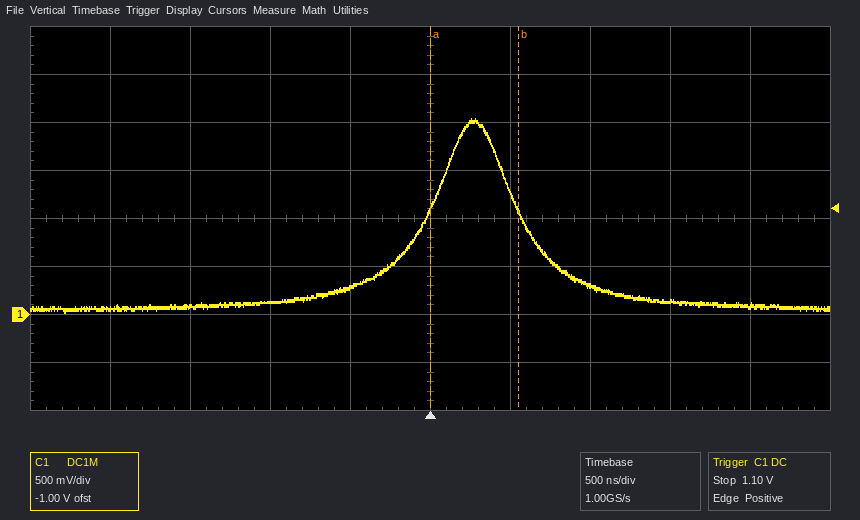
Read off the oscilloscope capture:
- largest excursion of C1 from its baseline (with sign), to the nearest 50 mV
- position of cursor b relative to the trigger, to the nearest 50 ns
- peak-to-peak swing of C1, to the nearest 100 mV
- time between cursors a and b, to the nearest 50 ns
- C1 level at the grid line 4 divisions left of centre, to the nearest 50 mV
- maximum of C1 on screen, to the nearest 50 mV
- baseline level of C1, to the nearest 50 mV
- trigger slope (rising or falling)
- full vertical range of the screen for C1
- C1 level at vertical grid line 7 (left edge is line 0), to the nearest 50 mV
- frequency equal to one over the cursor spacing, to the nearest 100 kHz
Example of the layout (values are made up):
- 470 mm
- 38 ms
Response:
- +1.95 V
- +550 ns
- 2.00 V
- 550 ns
- 50 mV
- 2.05 V
- 100 mV
- rising
- 4 V
- 300 mV
- 1.8 MHz
